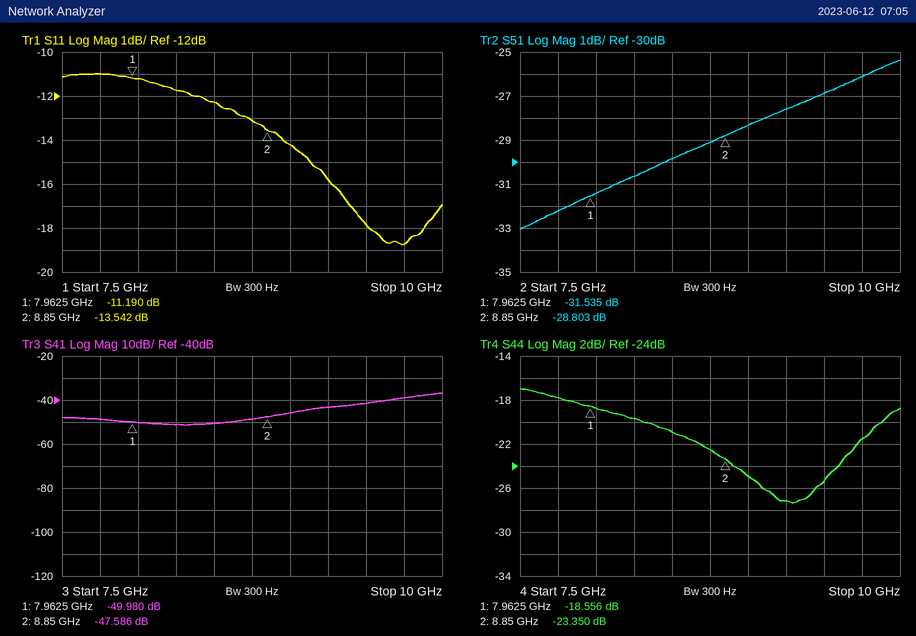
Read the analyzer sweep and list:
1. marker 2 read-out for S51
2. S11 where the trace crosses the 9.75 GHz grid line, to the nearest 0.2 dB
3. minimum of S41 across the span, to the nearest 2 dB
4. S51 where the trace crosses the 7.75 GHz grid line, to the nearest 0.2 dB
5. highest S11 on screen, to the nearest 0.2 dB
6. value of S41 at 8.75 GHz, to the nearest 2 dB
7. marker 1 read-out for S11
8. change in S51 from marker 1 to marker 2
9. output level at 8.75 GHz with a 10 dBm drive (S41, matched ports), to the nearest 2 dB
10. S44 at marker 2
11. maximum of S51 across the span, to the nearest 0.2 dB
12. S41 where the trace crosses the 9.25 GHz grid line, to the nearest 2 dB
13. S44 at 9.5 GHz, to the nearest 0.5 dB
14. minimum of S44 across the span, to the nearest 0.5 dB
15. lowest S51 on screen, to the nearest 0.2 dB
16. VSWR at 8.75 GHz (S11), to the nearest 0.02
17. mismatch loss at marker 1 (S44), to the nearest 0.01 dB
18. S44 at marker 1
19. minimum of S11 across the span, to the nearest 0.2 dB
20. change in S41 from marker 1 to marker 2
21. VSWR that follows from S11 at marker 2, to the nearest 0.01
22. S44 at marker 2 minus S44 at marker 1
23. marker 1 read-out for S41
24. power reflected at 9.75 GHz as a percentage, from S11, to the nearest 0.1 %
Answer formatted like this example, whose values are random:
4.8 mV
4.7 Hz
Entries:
-28.803 dB
-18.8 dB
-52 dB
-32.2 dB
-11.0 dB
-48 dB
-11.190 dB
2.732 dB
-38 dBm
-23.350 dB
-25.4 dB
-44 dB
-25.5 dB
-27.5 dB
-33.0 dB
1.56
0.06 dB
-18.556 dB
-18.8 dB
2.394 dB
1.53
-4.794 dB
-49.980 dB
1.3 %
